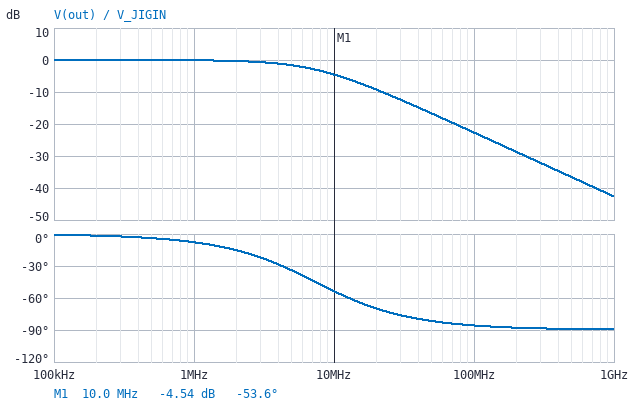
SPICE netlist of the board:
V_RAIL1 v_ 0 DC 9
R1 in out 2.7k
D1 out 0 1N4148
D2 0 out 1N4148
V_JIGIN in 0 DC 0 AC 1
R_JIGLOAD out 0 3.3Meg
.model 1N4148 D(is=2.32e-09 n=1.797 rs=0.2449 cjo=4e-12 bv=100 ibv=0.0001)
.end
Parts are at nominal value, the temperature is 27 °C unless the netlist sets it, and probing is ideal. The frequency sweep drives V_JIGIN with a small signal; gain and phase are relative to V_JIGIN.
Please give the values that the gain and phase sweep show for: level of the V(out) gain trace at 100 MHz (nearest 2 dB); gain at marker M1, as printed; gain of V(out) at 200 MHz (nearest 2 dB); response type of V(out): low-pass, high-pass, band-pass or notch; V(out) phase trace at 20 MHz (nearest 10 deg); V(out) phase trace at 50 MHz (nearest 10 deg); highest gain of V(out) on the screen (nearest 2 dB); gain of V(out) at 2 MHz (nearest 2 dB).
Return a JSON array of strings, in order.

["-22 dB", "-4.54 dB", "-28 dB", "low-pass", "-70 deg", "-80 deg", "0 dB", "0 dB"]
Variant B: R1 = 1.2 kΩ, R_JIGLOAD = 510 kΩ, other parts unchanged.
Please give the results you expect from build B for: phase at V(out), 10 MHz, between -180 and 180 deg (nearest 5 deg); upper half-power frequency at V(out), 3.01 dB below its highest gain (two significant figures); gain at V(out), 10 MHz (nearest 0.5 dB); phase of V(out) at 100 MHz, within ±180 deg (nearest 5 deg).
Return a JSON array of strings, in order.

["-30 deg", "17 MHz", "-1.5 dB", "-80 deg"]
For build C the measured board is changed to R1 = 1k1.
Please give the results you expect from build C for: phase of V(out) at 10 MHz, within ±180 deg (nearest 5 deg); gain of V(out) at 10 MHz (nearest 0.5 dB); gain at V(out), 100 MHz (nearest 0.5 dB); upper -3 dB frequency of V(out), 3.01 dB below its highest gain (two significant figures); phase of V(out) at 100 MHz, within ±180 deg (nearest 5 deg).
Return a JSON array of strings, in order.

["-30 deg", "-1.0 dB", "-15.0 dB", "18 MHz", "-80 deg"]
